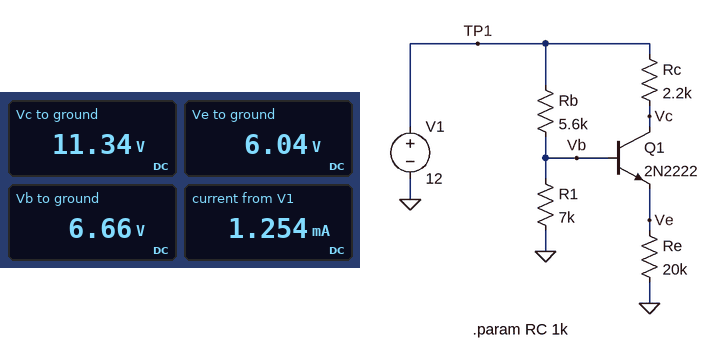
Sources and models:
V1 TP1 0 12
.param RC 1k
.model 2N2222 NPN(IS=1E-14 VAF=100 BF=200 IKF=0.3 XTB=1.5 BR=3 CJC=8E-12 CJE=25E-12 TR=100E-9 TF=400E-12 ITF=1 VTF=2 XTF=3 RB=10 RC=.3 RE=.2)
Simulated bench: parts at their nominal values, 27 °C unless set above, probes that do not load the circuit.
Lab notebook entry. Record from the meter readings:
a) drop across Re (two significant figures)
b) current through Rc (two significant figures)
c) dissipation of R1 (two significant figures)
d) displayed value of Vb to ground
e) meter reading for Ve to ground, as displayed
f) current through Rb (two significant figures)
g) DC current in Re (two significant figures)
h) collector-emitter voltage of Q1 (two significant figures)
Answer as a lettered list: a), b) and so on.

a) 6.0 V
b) 300 µA
c) 6.3 mW
d) 6.66 V
e) 6.04 V
f) 950 µA
g) 300 µA
h) 5.3 V
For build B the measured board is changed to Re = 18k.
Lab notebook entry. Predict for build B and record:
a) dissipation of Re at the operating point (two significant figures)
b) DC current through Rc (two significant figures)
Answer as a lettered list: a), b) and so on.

a) 2.0 mW
b) 330 µA
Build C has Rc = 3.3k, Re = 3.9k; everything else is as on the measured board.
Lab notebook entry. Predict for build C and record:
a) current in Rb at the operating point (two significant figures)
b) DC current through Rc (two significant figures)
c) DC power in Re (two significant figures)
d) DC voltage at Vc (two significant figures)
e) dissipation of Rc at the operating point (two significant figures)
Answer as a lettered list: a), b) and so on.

a) 960 µA
b) 1.5 mA
c) 9.2 mW
d) 7.0 V
e) 7.7 mW
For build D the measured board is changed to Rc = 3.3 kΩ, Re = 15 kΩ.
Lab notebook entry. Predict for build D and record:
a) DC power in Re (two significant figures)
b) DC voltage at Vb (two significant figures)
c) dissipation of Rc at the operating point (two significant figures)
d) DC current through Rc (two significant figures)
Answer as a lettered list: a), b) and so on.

a) 2.4 mW
b) 6.7 V
c) 530 µW
d) 400 µA
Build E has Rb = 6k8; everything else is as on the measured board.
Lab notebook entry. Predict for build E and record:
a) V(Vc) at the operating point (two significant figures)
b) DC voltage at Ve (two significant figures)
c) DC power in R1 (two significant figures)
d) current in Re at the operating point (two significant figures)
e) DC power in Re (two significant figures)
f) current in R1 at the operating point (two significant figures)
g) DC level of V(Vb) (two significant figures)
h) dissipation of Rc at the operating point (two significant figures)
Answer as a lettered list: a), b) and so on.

a) 11 V
b) 5.5 V
c) 5.3 mW
d) 270 µA
e) 1.5 mW
f) 870 µA
g) 6.1 V
h) 160 µW
